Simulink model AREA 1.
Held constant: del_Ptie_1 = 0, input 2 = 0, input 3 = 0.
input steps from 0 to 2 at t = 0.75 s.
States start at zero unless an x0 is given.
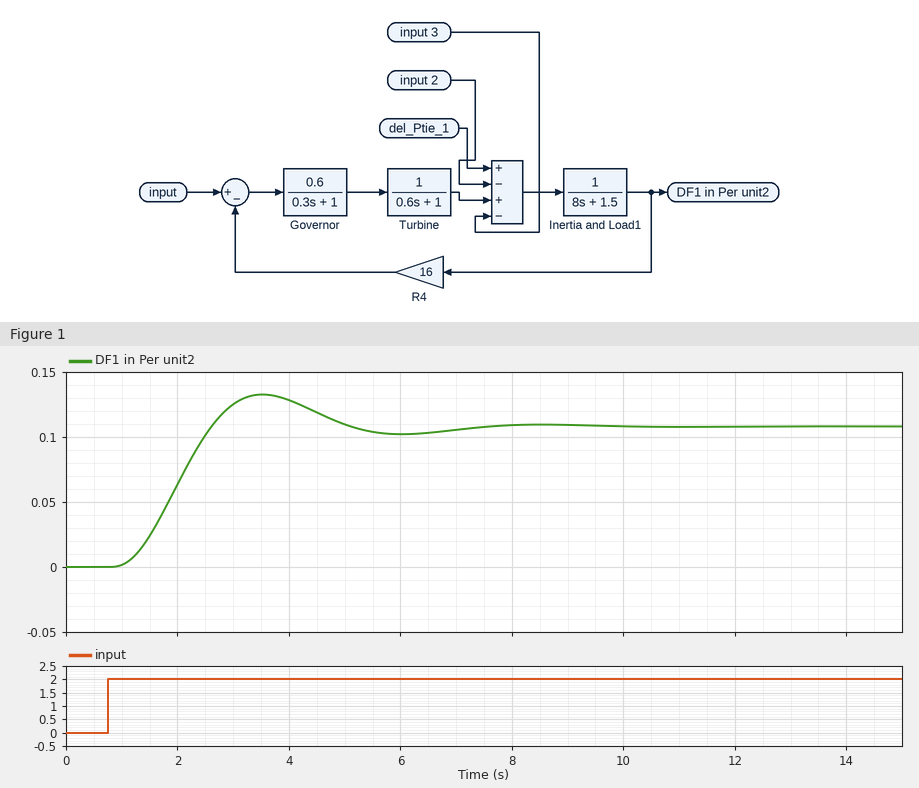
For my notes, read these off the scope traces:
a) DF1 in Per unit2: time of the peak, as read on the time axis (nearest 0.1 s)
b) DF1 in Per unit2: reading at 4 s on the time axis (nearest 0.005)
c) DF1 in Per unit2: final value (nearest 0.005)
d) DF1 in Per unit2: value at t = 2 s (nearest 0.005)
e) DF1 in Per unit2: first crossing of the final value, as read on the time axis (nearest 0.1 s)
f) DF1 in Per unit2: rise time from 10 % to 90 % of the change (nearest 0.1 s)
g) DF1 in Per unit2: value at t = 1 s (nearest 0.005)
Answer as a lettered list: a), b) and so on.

a) 3.5 s
b) 0.130
c) 0.110
d) 0.065
e) 2.6 s
f) 1.2 s
g) 0.000
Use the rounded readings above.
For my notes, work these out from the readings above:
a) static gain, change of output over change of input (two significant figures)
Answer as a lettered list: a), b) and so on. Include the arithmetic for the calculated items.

a) (0.11 - 0) / (2 - 0) = 0.055
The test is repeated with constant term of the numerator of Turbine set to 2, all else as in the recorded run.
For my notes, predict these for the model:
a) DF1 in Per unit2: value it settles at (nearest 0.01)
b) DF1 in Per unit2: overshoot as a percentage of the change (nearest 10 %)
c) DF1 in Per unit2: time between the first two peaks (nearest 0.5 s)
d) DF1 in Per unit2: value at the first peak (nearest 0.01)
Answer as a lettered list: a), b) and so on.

a) 0.12
b) 50 %
c) 3.5 s
d) 0.17
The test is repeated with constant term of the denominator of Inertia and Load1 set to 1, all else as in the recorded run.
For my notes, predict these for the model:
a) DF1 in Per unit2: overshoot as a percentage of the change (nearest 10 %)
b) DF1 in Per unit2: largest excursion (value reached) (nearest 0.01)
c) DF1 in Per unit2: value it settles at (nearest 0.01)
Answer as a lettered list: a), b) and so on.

a) 20 %
b) 0.14
c) 0.11
